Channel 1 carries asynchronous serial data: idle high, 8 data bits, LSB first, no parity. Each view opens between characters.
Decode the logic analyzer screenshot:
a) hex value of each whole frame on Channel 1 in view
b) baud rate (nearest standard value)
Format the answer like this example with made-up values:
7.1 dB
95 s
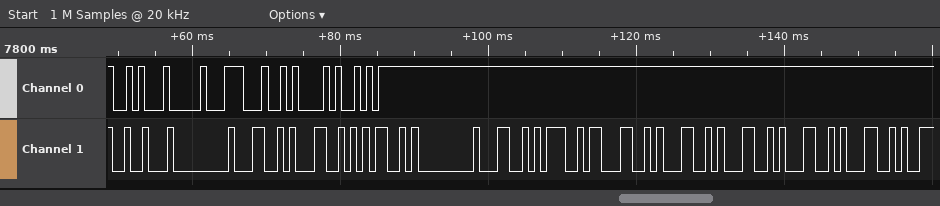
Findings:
12, 00, 4C, 4C, 4D, 00, 4C, A7, 4C, 4C, 4C, 4C, 4C
1200 baud
